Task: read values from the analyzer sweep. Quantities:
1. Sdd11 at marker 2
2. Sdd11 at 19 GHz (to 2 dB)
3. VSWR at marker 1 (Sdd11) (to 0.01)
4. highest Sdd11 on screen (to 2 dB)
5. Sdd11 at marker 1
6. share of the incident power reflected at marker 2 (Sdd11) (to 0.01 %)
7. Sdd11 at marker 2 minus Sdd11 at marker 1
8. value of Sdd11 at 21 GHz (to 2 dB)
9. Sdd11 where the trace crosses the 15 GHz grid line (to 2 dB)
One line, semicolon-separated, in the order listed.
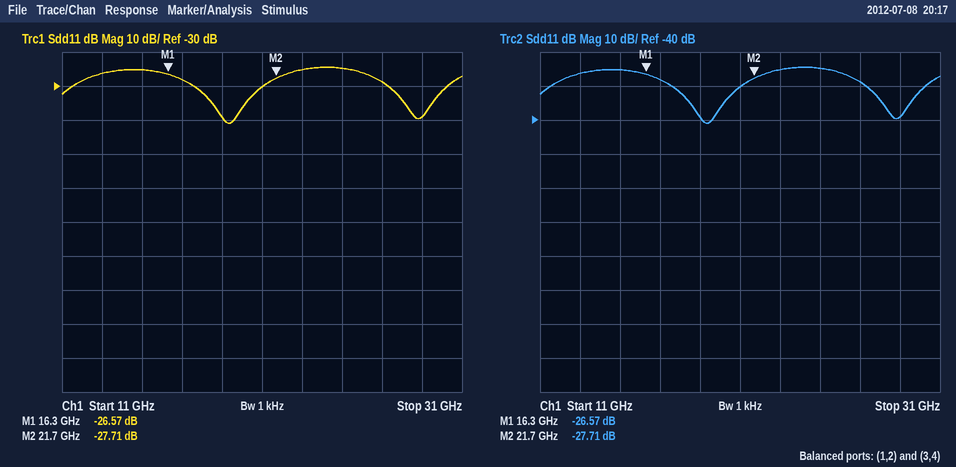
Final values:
-27.71 dB; -40 dB; 1.10; -24 dB; -26.57 dB; 0.17 %; -1.14 dB; -30 dB; -26 dB
